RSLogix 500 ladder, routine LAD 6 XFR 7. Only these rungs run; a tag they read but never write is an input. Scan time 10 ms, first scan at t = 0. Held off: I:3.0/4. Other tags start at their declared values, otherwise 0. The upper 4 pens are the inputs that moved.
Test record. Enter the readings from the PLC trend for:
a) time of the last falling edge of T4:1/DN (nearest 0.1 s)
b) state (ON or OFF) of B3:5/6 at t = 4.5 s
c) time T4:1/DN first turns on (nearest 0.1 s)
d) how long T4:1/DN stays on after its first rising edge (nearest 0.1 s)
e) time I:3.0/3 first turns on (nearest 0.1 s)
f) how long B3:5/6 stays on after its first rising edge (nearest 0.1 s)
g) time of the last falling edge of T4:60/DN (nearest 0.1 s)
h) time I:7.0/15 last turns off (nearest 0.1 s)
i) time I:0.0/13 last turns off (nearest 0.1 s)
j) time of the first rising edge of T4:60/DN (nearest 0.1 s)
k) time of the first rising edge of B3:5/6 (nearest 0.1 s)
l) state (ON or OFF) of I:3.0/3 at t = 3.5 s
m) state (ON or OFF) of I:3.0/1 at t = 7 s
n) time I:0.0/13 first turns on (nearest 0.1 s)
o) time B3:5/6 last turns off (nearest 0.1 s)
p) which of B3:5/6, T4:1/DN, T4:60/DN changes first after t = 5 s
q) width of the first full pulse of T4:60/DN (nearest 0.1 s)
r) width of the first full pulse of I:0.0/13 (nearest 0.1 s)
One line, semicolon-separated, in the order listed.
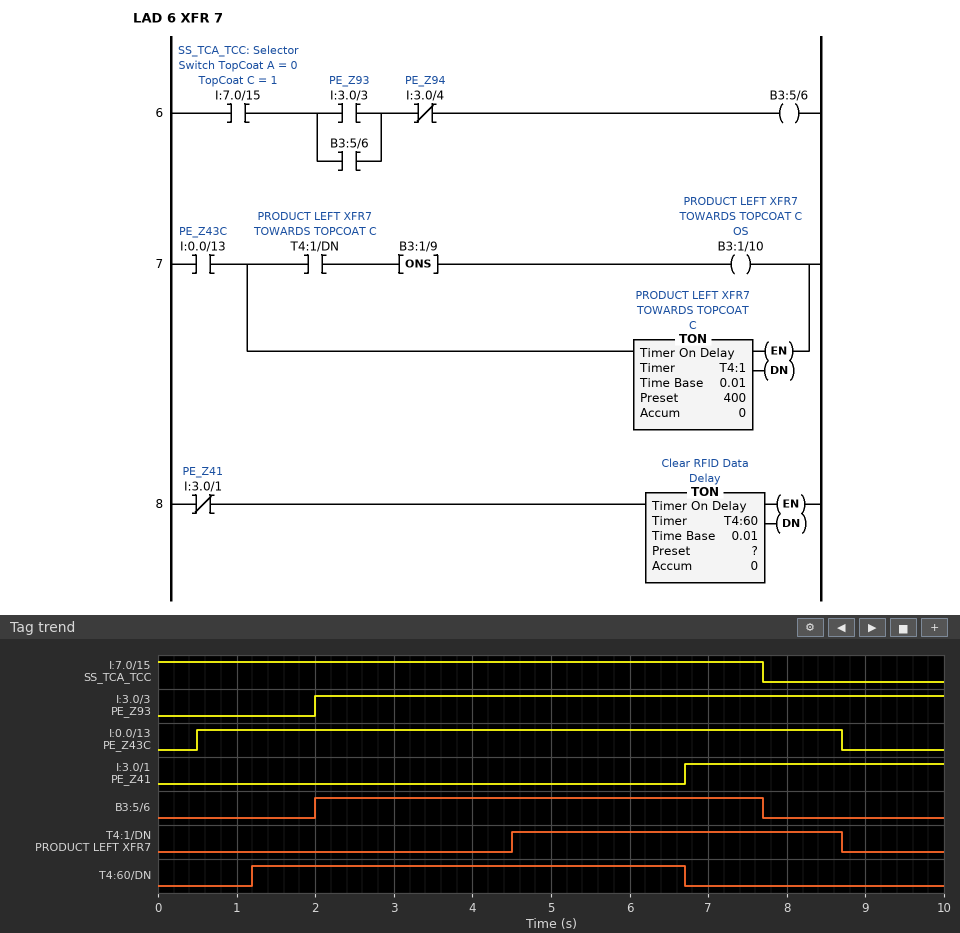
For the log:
8.7 s; ON; 4.5 s; 4.2 s; 2.0 s; 5.7 s; 6.7 s; 7.7 s; 8.7 s; 1.2 s; 2.0 s; ON; ON; 0.5 s; 7.7 s; T4:60/DN; 5.5 s; 8.2 s
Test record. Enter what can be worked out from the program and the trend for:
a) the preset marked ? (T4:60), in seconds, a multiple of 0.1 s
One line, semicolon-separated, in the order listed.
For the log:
1.2 s
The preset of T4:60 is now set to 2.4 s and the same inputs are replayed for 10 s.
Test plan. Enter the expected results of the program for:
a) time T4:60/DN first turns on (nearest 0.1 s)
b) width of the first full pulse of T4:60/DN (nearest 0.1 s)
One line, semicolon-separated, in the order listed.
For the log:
2.4 s; 4.3 s
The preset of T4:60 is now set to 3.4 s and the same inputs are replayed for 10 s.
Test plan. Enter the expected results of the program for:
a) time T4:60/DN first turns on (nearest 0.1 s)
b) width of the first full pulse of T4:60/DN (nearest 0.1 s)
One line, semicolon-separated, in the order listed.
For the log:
3.4 s; 3.3 s
